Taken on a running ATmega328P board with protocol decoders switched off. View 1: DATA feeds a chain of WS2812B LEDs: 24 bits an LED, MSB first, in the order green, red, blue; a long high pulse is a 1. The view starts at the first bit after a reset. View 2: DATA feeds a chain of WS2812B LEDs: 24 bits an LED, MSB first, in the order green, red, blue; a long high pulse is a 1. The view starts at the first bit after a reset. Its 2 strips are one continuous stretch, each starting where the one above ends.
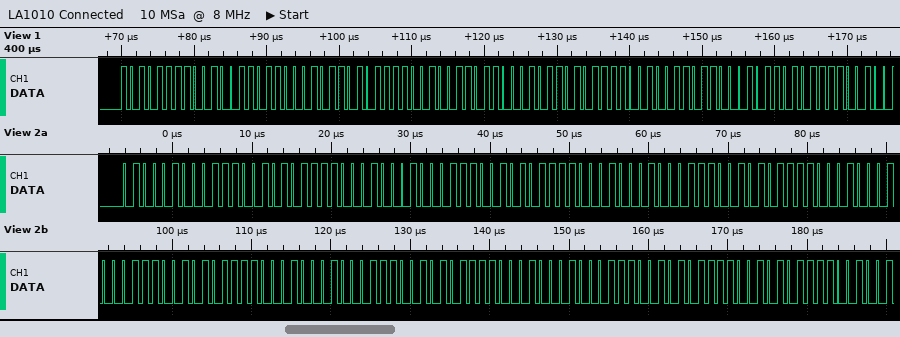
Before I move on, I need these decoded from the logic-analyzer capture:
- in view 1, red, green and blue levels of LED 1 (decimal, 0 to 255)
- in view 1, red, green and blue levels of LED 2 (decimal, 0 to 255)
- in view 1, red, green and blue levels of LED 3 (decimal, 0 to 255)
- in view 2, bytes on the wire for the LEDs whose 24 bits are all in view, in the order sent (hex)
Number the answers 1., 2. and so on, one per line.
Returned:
1. 38, 175, 197
2. 38, 175, 197
3. 38, 175, 197
4. 44 72 BC 44 72 BC 44 72 BC 44 72 BC 44 72 BC 44 72 BC
